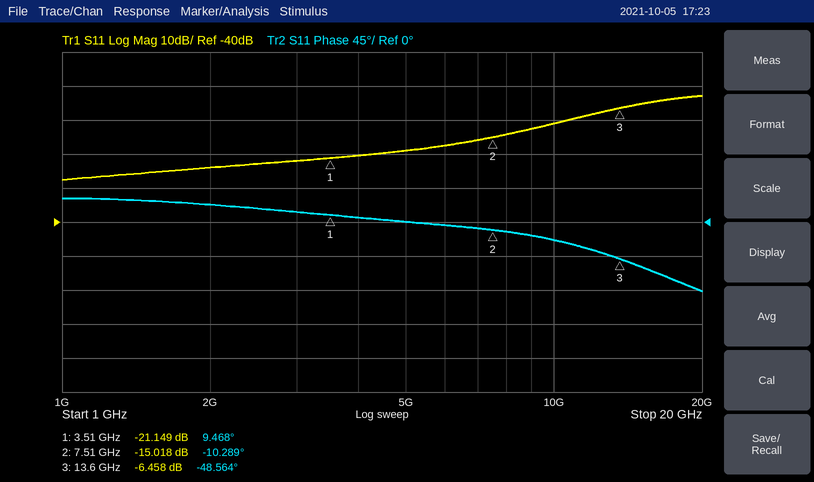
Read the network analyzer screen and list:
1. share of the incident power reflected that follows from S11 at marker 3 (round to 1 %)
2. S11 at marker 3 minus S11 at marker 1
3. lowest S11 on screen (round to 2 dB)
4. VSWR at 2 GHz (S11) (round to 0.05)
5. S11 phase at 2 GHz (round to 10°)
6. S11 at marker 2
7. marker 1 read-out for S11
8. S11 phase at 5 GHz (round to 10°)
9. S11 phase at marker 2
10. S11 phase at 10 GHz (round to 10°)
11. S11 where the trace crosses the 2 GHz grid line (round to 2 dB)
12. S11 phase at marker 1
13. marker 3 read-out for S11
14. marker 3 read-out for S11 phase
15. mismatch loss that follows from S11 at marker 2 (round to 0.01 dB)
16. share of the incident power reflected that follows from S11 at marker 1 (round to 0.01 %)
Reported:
23 %
14.691 dB
-28 dB
1.15
20°
-15.018 dB
-21.149 dB
0°
-10.289°
-20°
-24 dB
9.468°
-6.458 dB
-48.564°
0.14 dB
0.77 %
